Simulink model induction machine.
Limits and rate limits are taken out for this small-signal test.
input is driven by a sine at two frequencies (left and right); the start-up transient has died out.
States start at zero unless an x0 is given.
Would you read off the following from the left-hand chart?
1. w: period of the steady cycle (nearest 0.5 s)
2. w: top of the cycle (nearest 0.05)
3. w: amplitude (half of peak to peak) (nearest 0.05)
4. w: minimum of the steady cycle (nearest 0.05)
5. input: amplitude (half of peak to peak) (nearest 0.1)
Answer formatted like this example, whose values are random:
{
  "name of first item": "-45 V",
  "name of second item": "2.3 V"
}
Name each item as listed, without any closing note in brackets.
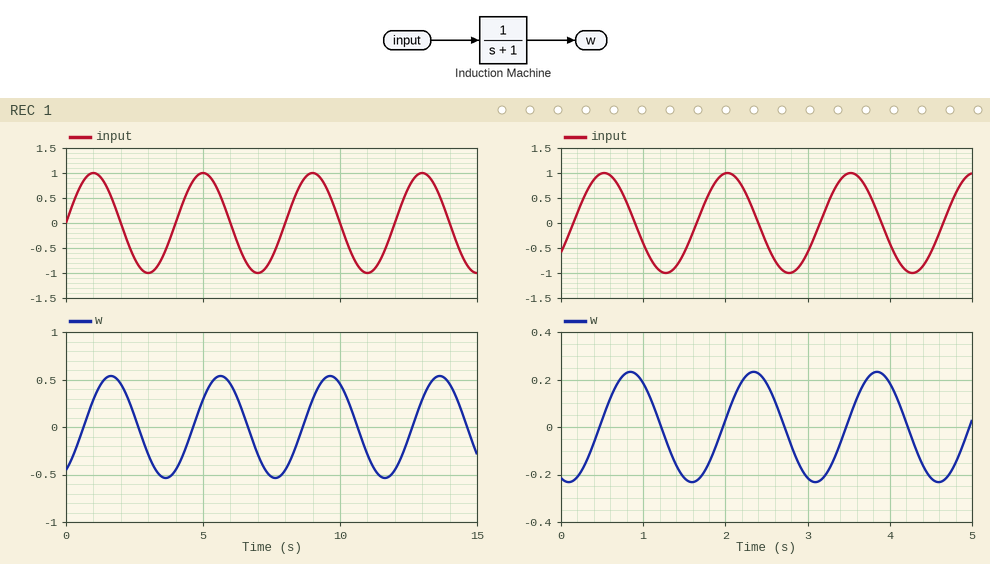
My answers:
{
  "w: period of the steady cycle": "4.0 s",
  "w: top of the cycle": "0.55",
  "w: amplitude (half of peak to peak)": "0.55",
  "w: minimum of the steady cycle": "-0.55",
  "input: amplitude (half of peak to peak)": "1.0"
}
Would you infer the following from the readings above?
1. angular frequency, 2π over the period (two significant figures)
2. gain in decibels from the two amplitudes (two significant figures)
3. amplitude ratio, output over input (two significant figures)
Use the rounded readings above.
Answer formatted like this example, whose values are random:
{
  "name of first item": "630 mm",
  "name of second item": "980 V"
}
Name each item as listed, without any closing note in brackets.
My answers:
{
  "angular frequency, 2π over the period": "1.6 rad/s",
  "gain in decibels from the two amplitudes": "-5.2 dB",
  "amplitude ratio, output over input": "0.55"
}
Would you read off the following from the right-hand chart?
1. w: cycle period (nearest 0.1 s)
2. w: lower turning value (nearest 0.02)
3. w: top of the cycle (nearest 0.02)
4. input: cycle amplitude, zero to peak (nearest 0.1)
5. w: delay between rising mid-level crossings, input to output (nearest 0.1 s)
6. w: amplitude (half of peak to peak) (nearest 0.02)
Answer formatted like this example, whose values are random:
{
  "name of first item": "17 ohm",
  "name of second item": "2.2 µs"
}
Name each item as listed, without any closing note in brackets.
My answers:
{
  "w: cycle period": "1.5 s",
  "w: lower turning value": "-0.24",
  "w: top of the cycle": "0.24",
  "input: cycle amplitude, zero to peak": "1.0",
  "w: delay between rising mid-level crossings, input to output": "0.3 s",
  "w: amplitude (half of peak to peak)": "0.24"
}
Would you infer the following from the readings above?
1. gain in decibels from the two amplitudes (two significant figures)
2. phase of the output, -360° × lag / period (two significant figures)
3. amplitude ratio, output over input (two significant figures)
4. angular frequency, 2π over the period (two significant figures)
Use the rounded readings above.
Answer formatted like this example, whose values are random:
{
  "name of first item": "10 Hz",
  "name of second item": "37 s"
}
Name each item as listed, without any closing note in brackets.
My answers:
{
  "gain in decibels from the two amplitudes": "-12 dB",
  "phase of the output, -360° × lag / period": "-72°",
  "amplitude ratio, output over input": "0.24",
  "angular frequency, 2π over the period": "4.2 rad/s"
}
